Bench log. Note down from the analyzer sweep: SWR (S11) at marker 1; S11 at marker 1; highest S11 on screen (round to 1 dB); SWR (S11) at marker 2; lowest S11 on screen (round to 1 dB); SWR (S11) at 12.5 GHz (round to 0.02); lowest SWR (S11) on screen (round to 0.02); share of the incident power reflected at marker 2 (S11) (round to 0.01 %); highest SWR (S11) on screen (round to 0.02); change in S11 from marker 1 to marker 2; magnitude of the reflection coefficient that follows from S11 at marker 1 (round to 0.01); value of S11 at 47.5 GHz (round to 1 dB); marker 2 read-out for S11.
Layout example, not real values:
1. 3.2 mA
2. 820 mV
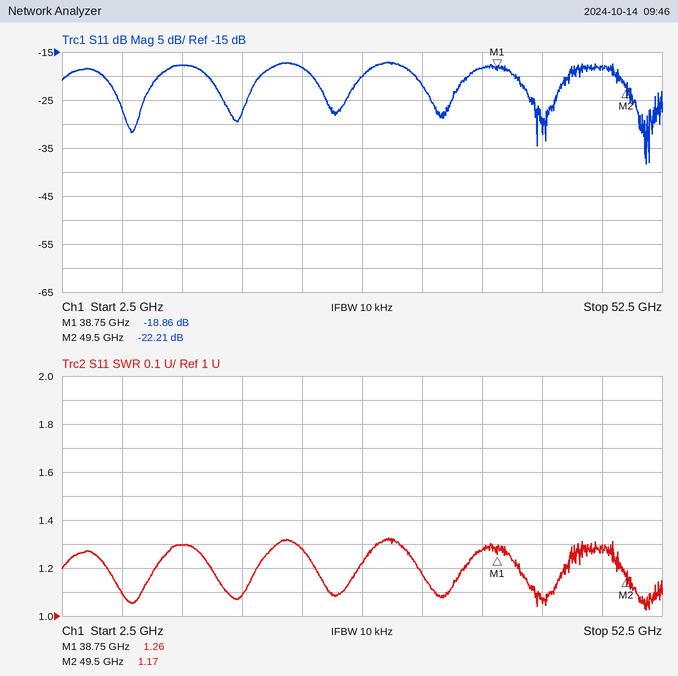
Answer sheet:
1. 1.26
2. -18.86 dB
3. -17 dB
4. 1.17
5. -38 dB
6. 1.30
7. 1.02
8. 0.60 %
9. 1.32
10. -3.35 dB
11. 0.11
12. -18 dB
13. -22.21 dB
